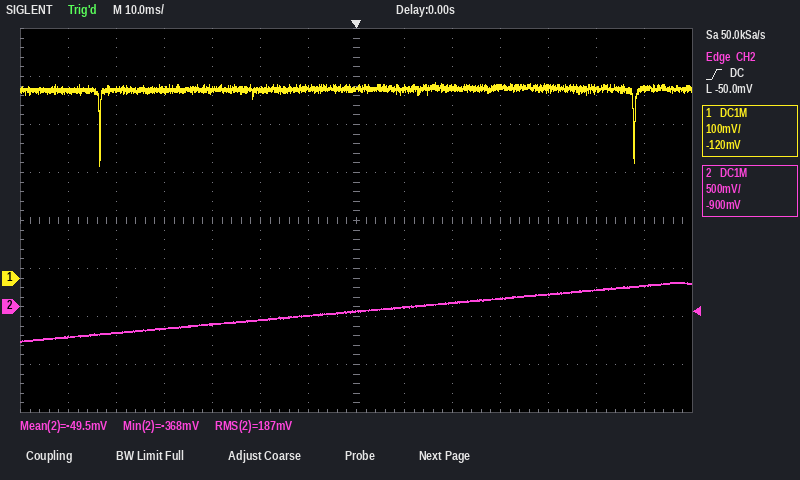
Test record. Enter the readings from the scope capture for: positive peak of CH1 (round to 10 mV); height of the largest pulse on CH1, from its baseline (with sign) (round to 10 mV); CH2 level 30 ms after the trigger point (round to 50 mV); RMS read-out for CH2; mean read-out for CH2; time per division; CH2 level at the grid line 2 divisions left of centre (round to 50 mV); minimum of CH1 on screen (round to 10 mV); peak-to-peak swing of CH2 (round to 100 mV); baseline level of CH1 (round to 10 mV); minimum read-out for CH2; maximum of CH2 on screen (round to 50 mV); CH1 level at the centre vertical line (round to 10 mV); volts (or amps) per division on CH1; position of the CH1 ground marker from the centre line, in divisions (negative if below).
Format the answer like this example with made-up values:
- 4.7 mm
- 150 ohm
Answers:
- 410 mV
- -160 mV
- 100 mV
- 187 mV
- -49.5 mV
- 10 ms
- -150 mV
- 230 mV
- 600 mV
- 390 mV
- -368 mV
- 250 mV
- 390 mV
- 100 mV
- -1.2 div
